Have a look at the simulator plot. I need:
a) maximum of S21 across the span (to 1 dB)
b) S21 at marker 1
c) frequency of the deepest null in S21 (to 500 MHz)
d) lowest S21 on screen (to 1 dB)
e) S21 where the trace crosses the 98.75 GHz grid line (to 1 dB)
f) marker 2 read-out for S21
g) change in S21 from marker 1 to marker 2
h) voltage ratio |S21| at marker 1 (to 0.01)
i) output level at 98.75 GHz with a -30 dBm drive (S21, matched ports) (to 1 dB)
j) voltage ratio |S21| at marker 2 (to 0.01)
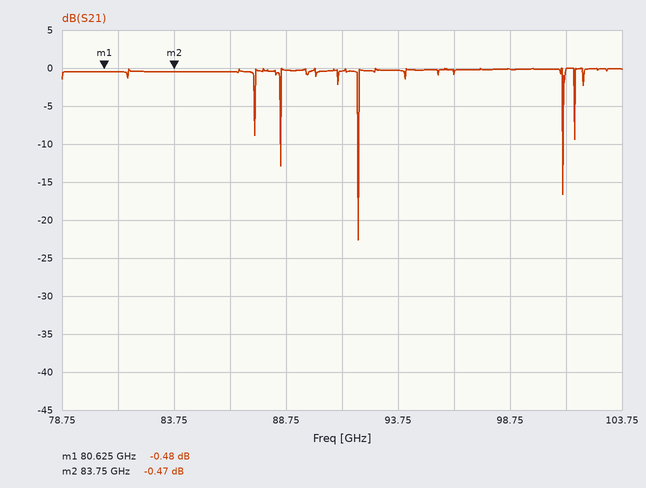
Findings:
0 dB
-0.48 dB
92.0 GHz
-23 dB
0 dB
-0.47 dB
0.01 dB
0.95
-30 dBm
0.95
